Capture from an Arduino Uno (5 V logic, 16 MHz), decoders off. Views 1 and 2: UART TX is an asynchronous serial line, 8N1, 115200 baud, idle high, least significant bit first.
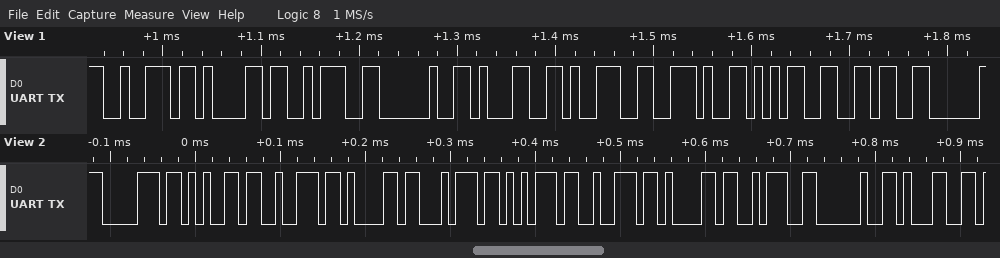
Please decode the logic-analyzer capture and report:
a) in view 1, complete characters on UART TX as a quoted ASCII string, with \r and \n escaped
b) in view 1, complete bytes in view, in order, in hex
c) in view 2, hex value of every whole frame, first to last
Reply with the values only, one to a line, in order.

"ra: 19.56"
72 61 3A 20 31 39 2E 35 36
70 65 72 61 74 75 72 61 3A 20 31
